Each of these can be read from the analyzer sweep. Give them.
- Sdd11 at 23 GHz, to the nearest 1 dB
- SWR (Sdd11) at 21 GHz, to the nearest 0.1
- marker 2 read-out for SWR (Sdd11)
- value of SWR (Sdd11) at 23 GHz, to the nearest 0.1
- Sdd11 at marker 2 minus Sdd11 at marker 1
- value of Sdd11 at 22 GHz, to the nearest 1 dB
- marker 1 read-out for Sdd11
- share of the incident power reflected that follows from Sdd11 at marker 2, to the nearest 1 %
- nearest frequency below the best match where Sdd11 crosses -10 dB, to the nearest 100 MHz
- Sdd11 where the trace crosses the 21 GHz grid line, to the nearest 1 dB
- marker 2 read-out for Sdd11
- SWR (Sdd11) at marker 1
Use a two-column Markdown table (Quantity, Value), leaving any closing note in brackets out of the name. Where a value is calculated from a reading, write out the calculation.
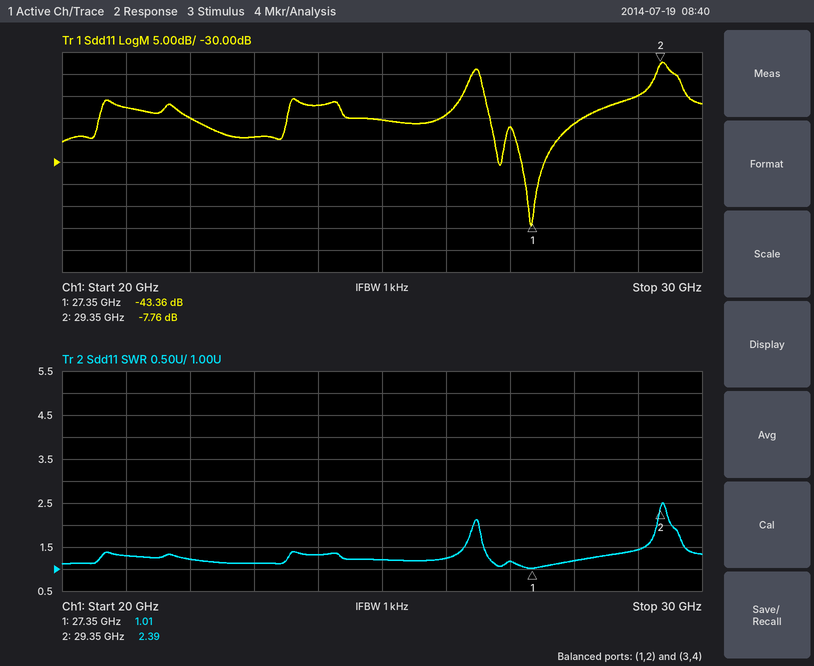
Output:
| Quantity | Value |
|---|---|
| Sdd11 at 23 GHz, to the nearest 1 dB | -24 dB |
| SWR (Sdd11) at 21 GHz, to the nearest 0.1 | 1.3 |
| marker 2 read-out for SWR | 2.39 |
| value of SWR (Sdd11) at 23 GHz, to the nearest 0.1 | 1.1 |
| Sdd11 at marker 2 minus Sdd11 at marker 1 | -7.76 − (-43.36) = 35.60 dB |
| value of Sdd11 at 22 GHz, to the nearest 1 dB | -20 dB |
| marker 1 read-out for Sdd11 | -43.36 dB |
| share of the incident power reflected that follows from Sdd11 at marker 2, to the nearest 1 % | 10^(-7.76/10) ≈ 17 % |
| nearest frequency below the best match where Sdd11 crosses -10 dB, to the nearest 100 MHz | 26.5 GHz |
| Sdd11 where the trace crosses the 21 GHz grid line, to the nearest 1 dB | -18 dB |
| marker 2 read-out for Sdd11 | -7.76 dB |
| SWR (Sdd11) at marker 1 | 1.01 |
